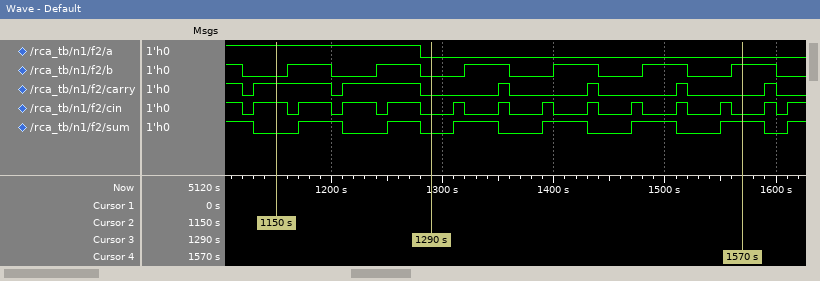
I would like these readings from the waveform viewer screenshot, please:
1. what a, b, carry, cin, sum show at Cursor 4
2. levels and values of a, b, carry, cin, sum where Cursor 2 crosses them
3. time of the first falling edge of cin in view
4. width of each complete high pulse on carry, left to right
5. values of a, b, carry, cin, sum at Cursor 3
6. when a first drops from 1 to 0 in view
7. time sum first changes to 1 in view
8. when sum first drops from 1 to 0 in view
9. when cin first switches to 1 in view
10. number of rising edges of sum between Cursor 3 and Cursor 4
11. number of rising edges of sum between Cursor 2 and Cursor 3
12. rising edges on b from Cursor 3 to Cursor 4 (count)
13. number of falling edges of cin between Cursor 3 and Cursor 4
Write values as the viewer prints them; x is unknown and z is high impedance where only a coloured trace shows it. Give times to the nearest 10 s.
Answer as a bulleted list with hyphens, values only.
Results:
- a=0, b=1, carry=0, cin=0, sum=1
- a=1, b=0, carry=1, cin=1, sum=0
- 1120 s
- 70 s, 70 s, 10 s, 10 s, 10 s, 10 s
- a=0, b=0, carry=0, cin=0, sum=0
- 1280 s
- 1170 s
- 1130 s
- 1130 s
- 4
- 2
- 4
- 7
